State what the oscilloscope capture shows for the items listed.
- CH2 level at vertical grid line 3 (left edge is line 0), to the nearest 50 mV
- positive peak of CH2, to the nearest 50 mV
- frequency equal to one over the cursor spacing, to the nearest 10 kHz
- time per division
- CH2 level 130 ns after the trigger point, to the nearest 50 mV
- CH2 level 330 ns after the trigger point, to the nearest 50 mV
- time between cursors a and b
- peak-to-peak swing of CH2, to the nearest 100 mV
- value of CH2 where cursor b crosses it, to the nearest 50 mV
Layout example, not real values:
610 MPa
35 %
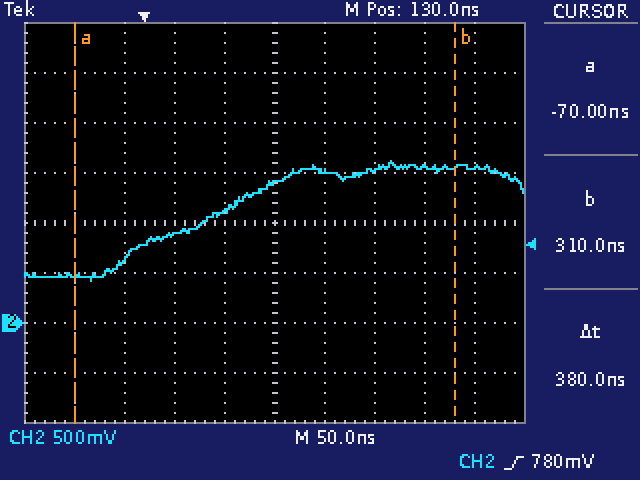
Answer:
900 mV
1.60 V
2.63 MHz
50 ns
1.40 V
1.55 V
380 ns
1.20 V
1.55 V
